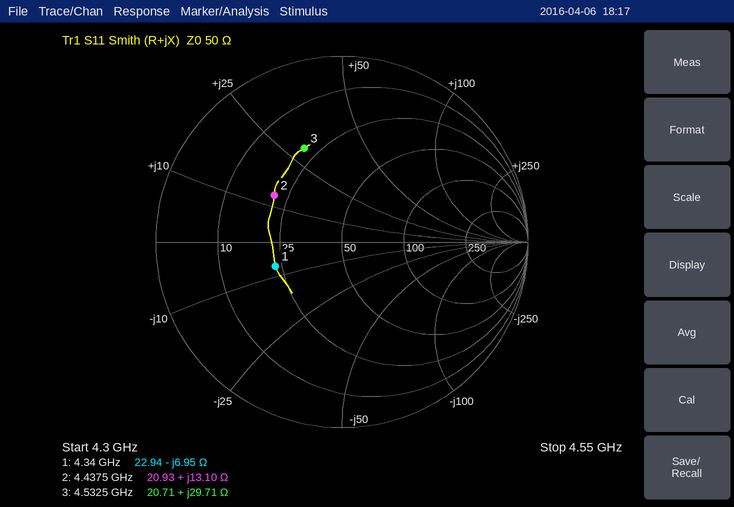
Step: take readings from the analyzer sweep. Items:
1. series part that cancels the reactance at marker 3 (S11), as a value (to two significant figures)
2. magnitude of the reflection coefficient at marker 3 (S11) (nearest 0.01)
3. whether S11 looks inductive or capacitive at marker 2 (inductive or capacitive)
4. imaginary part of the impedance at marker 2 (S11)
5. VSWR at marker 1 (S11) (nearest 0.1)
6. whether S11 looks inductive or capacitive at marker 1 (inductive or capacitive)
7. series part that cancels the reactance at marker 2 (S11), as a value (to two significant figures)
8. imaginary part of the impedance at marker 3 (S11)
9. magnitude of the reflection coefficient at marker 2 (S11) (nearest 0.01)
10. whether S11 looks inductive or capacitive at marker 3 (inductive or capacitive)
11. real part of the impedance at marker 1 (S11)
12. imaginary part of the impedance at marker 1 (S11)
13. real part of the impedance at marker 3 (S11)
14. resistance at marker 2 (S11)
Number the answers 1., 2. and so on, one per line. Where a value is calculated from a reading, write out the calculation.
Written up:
1. C = 1/(2π × 4.5325 GHz × 29.71 Ω) ≈ 1.2 pF
2. 0.54
3. inductive
4. +13.10 Ω
5. 2.2
6. capacitive
7. C = 1/(2π × 4.4375 GHz × 13.1 Ω) ≈ 2.7 pF
8. +29.71 Ω
9. 0.44
10. inductive
11. 22.94 Ω
12. -6.95 Ω
13. 20.71 Ω
14. 20.93 Ω
